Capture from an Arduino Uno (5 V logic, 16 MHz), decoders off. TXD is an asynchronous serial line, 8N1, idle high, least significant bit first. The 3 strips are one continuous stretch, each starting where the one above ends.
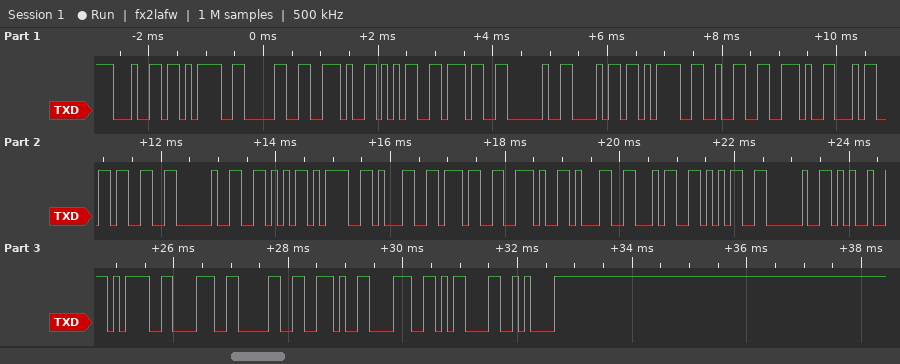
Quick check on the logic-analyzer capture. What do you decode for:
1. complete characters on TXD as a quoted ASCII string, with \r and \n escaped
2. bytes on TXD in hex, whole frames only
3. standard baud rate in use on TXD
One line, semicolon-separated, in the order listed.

"d=0.57 h=2.43 V=17.145 %=80.8\r\n"; 64 3D 30 2E 35 37 20 68 3D 32 2E 34 33 20 56 3D 31 37 2E 31 34 35 20 25 3D 38 30 2E 38 0D 0A; 9600 baud
